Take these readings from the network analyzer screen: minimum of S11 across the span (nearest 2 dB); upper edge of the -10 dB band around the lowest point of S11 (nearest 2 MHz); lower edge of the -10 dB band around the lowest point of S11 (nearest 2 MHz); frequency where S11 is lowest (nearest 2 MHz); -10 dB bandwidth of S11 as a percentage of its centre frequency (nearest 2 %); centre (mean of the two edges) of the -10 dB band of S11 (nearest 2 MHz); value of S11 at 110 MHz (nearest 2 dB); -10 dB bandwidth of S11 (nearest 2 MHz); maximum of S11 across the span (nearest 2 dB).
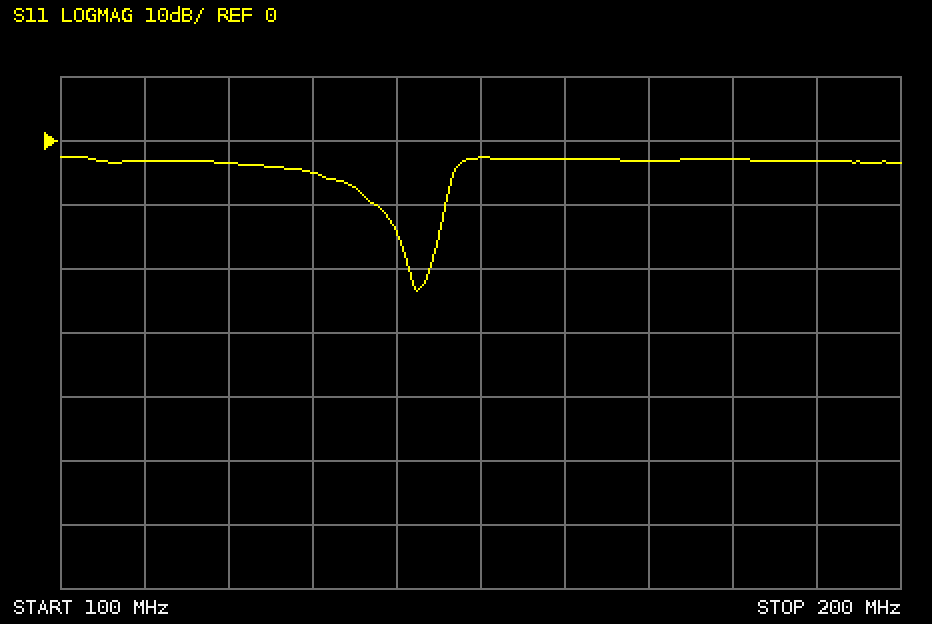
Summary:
-24 dB
146 MHz
138 MHz
142 MHz
6 %
142 MHz
-4 dB
8 MHz
-2 dB
